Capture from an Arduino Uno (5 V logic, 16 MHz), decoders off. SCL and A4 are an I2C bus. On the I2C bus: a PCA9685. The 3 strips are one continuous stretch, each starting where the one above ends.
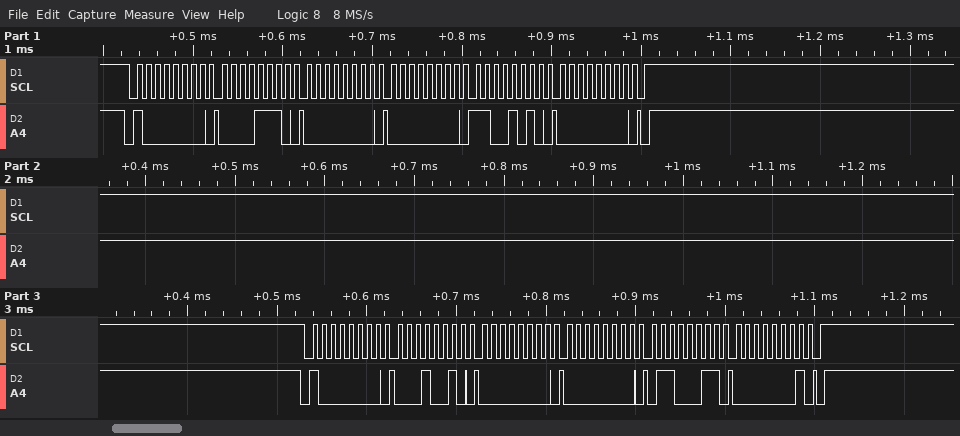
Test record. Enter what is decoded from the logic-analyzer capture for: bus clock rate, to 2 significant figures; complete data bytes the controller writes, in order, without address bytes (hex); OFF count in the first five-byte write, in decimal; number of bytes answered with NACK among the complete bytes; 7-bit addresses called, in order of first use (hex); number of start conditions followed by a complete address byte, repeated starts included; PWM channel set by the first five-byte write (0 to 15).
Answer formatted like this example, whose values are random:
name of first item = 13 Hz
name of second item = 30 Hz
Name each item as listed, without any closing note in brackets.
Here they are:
bus clock rate, to 2 significant figures = 100 kHz
complete data bytes the controller writes, in order, without address bytes = 0E 00 00 CA 00 12 00 00 63 01
OFF count in the first five-byte write, in decimal = 202
number of bytes answered with NACK among the complete bytes = 0
7-bit addresses called, in order of first use = 0x40
number of start conditions followed by a complete address byte, repeated starts included = 2
PWM channel set by the first five-byte write = 2
